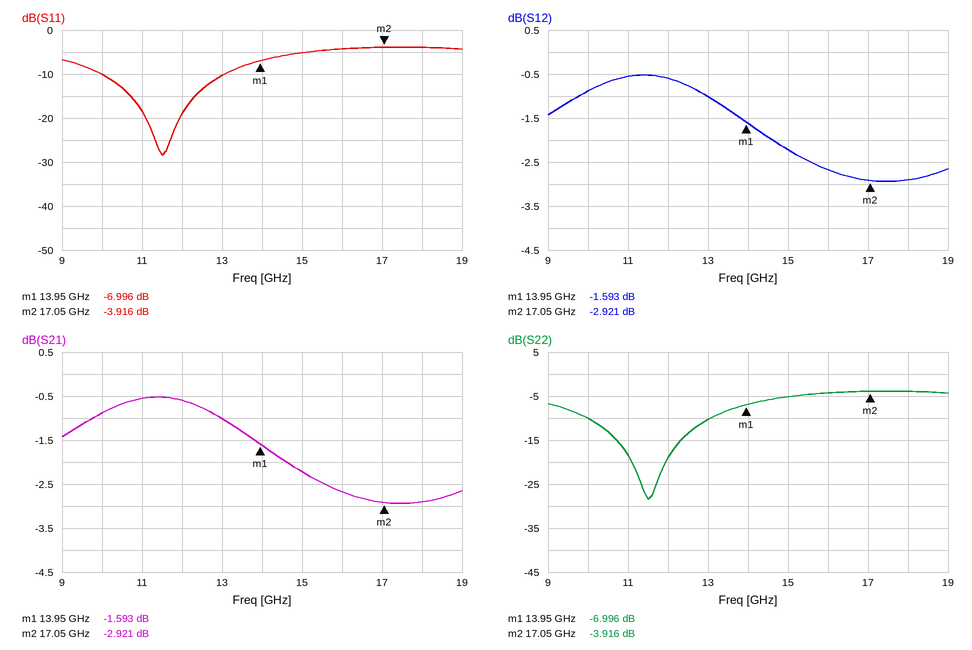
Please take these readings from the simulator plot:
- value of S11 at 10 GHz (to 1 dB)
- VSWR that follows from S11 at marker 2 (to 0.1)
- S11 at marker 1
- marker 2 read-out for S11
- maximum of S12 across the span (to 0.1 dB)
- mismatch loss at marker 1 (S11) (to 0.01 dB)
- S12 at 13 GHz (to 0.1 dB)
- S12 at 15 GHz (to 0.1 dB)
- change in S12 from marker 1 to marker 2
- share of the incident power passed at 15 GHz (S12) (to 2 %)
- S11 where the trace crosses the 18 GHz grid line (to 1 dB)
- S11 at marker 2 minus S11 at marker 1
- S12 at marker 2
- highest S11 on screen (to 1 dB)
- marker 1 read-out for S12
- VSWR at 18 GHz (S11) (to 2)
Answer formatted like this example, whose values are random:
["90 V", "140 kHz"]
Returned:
["-10 dB", "4.5", "-6.996 dB", "-3.916 dB", "-0.5 dB", "0.97 dB", "-1.0 dB", "-2.2 dB", "-1.328 dB", "60 %", "-4 dB", "3.080 dB", "-2.921 dB", "-4 dB", "-1.593 dB", "4"]
